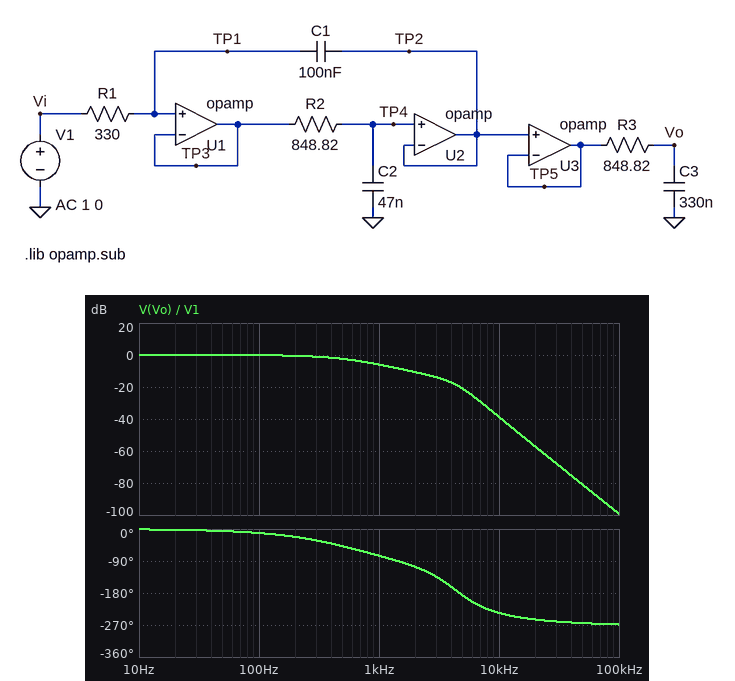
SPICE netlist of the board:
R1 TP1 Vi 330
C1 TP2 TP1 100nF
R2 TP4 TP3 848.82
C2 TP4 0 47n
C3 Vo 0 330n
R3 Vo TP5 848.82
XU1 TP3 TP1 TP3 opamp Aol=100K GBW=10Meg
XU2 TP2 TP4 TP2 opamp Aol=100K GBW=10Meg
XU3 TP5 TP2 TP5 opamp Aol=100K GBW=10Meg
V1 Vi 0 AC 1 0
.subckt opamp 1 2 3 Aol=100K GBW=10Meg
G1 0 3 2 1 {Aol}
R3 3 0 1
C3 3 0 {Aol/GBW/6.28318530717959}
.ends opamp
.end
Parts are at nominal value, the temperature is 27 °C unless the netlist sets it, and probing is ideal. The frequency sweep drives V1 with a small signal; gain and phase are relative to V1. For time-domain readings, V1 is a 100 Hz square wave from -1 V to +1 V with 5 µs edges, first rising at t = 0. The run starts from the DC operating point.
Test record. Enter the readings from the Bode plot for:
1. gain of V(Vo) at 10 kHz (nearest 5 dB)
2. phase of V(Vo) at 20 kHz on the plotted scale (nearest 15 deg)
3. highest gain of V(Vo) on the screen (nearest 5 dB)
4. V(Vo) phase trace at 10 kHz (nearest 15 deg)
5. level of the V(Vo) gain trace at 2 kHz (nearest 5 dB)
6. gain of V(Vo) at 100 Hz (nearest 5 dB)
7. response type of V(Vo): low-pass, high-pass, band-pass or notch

-40 dB
-255 deg
0 dB
-240 deg
-10 dB
0 dB
low-pass
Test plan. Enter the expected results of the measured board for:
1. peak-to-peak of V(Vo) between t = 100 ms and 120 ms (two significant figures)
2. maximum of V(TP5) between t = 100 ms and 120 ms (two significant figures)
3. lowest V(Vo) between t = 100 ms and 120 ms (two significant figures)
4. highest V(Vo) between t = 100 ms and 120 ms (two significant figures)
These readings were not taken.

2.0 V
1.3 V
-1.0 V
1.0 V
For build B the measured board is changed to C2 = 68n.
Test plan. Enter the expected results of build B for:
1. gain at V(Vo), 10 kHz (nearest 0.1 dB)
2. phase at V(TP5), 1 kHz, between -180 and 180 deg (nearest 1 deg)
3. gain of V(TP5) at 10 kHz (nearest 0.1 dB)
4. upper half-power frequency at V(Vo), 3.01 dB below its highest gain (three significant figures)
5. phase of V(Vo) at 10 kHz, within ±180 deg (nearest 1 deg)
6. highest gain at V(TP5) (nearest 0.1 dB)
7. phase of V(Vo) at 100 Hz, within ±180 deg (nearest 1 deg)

-42.4 dB
-21 deg
-17.5 dB
571 Hz
122 deg
0.1 dB
-12 deg
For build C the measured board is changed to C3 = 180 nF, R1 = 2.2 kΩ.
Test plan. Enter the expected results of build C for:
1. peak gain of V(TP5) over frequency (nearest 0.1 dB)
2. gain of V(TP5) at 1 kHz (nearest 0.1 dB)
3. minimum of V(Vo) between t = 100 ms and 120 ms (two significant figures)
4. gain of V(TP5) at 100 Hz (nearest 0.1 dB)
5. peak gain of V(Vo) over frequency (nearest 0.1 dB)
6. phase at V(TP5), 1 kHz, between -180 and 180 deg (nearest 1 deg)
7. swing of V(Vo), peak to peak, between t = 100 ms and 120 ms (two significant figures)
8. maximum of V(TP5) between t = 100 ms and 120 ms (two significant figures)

7.6 dB
3.1 dB
-1.3 V
0 dB
2.4 dB
-21 deg
2.7 V
2.0 V
